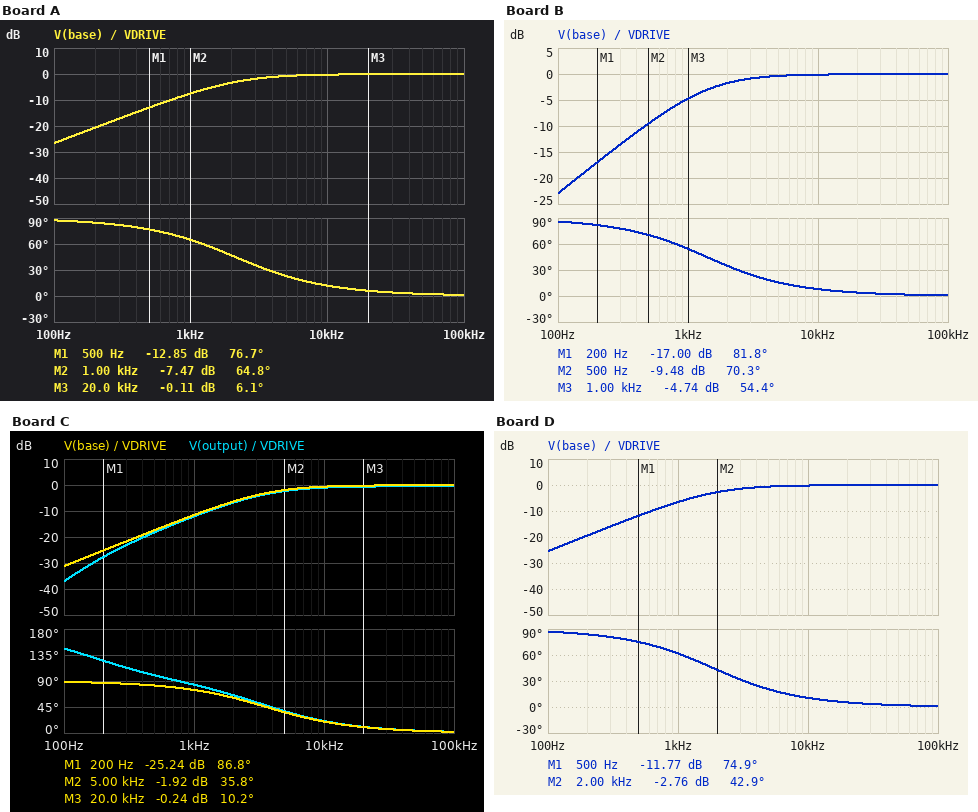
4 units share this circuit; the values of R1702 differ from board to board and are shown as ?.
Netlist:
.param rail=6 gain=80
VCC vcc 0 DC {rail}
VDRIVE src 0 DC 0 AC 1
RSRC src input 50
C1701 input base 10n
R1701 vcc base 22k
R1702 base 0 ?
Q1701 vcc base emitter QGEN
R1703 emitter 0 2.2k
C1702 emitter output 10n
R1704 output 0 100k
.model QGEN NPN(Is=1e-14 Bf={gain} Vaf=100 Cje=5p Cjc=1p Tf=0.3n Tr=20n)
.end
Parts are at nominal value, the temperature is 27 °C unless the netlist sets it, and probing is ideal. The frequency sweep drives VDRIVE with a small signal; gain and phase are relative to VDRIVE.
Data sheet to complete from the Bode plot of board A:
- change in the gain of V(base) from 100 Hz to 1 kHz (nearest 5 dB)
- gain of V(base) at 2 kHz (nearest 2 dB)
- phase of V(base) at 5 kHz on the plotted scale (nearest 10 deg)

20 dB
-4 dB
20 deg
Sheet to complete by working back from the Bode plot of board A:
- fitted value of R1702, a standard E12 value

12 kΩ
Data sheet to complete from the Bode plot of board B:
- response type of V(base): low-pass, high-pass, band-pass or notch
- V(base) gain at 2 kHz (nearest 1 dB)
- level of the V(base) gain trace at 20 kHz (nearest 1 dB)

high-pass
-2 dB
0 dB
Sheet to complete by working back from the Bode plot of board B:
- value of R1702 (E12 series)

27 kΩ
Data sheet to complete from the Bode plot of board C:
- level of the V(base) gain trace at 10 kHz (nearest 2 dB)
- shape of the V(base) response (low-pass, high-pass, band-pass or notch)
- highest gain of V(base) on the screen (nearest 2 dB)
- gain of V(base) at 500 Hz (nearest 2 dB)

0 dB
high-pass
0 dB
-18 dB
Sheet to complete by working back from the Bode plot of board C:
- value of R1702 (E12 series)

5.6 kΩ
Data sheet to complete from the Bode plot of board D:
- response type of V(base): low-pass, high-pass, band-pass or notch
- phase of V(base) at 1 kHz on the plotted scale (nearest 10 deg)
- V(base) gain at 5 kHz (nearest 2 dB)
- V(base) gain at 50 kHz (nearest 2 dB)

high-pass
60 deg
0 dB
0 dB
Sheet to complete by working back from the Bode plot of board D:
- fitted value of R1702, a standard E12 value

15 kΩ
